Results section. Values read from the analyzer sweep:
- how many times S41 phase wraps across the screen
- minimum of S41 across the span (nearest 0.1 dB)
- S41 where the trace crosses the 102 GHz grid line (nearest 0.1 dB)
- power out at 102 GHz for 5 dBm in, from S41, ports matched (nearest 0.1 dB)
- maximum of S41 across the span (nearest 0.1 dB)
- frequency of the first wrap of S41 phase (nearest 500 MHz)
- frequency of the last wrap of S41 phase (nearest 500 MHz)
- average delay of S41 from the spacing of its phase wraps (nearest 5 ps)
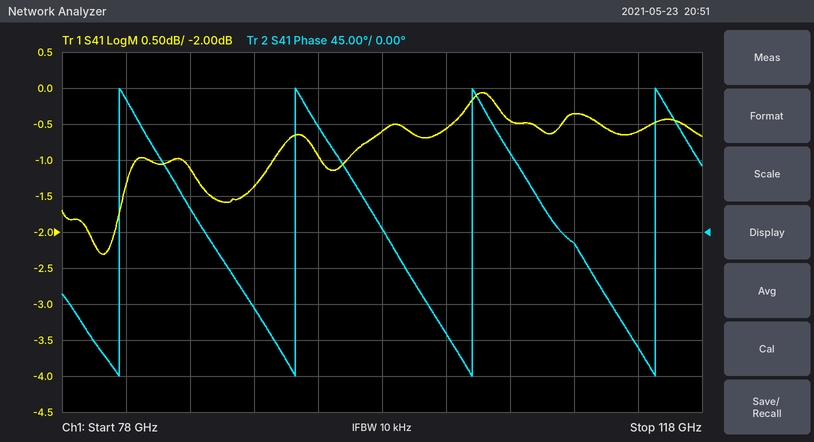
4
-2.3 dB
-0.6 dB
4.4 dBm
-0.1 dB
81.5 GHz
115.0 GHz
90 ps
